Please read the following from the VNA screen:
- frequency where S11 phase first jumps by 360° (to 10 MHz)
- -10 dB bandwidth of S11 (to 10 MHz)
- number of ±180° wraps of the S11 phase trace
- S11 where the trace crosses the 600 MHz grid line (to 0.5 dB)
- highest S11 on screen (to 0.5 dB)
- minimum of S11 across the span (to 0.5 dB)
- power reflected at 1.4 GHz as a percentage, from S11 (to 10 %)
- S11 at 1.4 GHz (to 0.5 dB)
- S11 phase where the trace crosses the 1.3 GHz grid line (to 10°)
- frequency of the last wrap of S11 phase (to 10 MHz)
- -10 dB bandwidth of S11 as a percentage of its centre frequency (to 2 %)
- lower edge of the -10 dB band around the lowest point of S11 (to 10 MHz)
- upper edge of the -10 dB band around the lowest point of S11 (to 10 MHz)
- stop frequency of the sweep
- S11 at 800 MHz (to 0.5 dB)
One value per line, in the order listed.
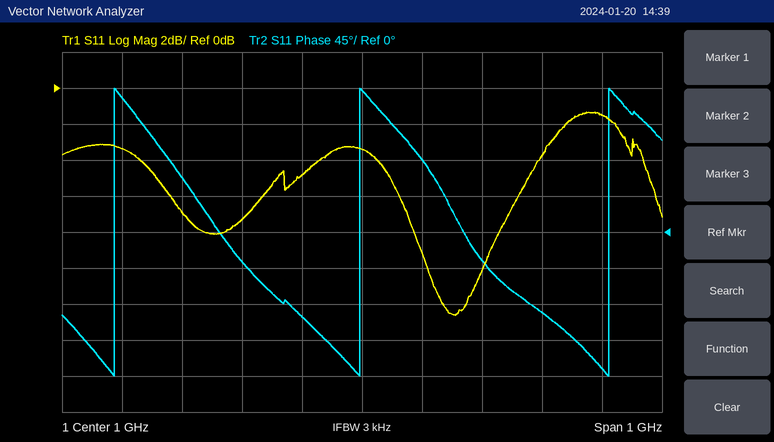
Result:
590 MHz
90 MHz
3
-3.5 dB
-1.5 dB
-12.5 dB
70 %
-1.5 dB
-100°
1.41 GHz
8 %
1.11 GHz
1.20 GHz
1.5 GHz
-7.5 dB
